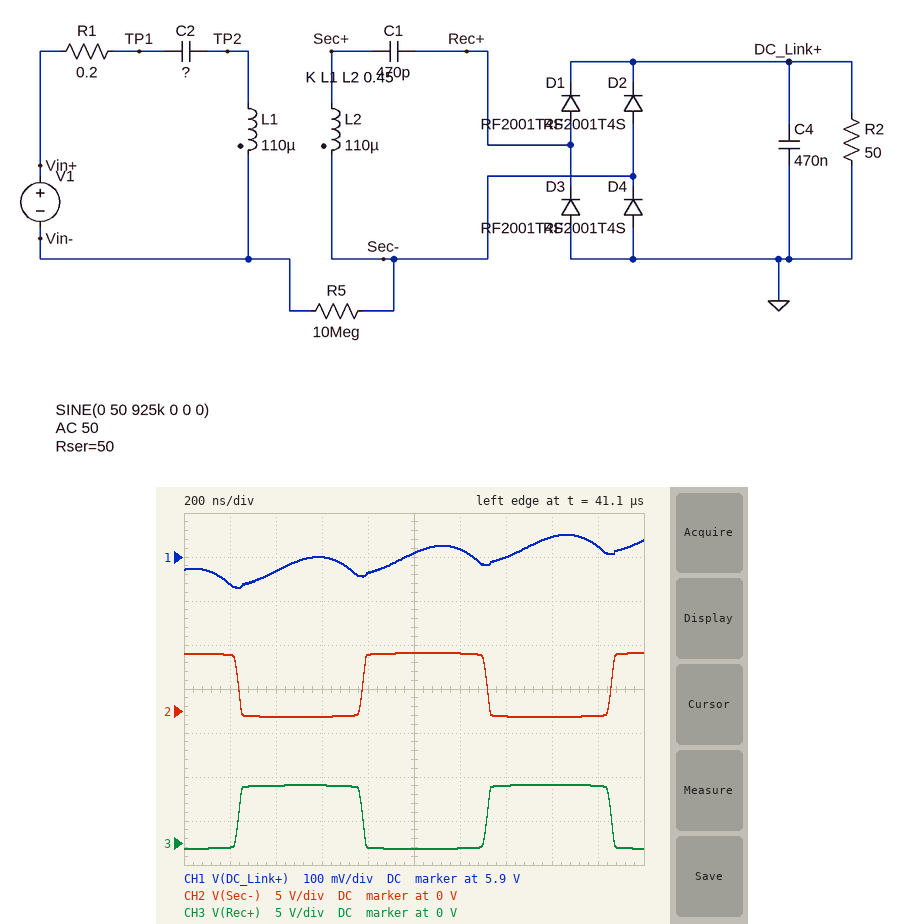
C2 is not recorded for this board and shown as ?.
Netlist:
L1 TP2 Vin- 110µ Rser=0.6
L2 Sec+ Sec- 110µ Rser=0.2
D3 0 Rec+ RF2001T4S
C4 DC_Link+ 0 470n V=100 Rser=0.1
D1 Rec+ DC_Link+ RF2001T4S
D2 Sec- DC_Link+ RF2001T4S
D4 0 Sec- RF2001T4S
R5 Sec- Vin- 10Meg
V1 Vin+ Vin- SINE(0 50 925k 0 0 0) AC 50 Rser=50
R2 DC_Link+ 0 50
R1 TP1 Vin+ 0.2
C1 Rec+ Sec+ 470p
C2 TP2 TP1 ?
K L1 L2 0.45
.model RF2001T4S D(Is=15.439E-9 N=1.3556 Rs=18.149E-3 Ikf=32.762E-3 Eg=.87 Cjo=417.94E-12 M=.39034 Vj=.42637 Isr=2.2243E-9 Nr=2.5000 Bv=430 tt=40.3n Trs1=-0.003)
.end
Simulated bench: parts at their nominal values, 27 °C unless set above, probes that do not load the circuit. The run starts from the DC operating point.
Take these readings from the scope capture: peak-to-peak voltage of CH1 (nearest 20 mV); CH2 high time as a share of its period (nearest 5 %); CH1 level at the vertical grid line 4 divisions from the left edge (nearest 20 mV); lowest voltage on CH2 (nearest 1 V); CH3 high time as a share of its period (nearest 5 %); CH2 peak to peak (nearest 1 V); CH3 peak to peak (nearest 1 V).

120 mV
50 %
5.86 V
-1 V
50 %
7 V
7 V
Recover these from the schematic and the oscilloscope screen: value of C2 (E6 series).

1.5 nF
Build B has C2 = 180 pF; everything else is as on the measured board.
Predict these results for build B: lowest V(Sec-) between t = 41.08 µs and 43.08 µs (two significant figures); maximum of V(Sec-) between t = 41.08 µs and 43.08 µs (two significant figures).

-600 mV
2.7 V
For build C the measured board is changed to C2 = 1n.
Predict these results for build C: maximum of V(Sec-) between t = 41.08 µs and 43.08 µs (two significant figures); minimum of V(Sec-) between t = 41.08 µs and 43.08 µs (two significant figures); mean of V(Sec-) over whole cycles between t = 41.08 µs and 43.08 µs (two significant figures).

8.3 V
-680 mV
3.8 V
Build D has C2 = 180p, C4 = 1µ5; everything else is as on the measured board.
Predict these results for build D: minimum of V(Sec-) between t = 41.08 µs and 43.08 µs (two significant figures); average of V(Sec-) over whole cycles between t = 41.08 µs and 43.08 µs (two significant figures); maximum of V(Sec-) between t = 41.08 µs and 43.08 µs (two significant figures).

-600 mV
550 mV
1.7 V
